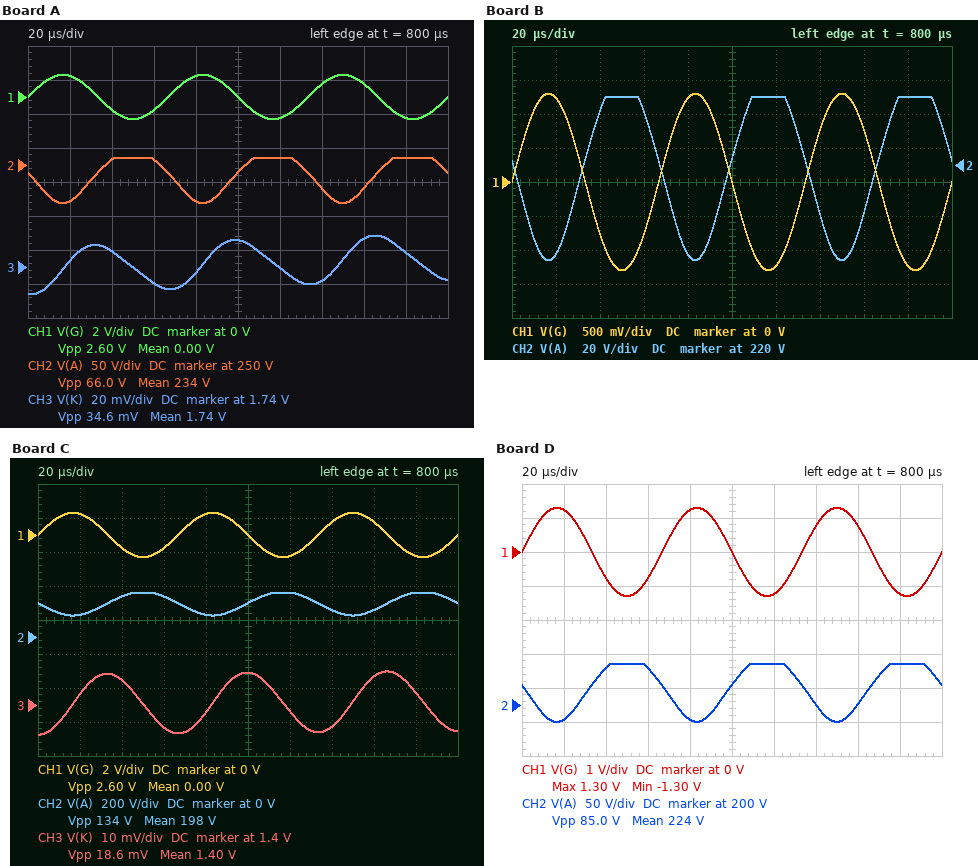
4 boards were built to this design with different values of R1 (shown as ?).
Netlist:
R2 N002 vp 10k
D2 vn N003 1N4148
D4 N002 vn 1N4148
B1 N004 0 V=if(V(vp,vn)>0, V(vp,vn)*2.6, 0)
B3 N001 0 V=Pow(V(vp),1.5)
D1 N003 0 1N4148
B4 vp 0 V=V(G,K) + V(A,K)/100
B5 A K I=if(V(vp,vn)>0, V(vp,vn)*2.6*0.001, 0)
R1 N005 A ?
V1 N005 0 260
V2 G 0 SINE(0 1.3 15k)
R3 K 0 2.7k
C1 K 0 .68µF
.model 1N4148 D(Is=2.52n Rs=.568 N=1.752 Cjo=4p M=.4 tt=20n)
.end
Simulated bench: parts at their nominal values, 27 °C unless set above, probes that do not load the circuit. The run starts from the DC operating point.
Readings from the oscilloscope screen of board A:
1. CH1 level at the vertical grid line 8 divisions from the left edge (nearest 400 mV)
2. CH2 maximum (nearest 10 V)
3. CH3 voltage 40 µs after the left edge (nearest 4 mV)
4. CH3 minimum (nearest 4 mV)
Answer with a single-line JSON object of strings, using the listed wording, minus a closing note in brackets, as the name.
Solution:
{"CH1 level at the vertical grid line 8 divisions from the left edge": "800 mV", "CH2 maximum": "260 V", "CH3 voltage 40 µs after the left edge": "1.748 V", "CH3 minimum": "1.724 V"}
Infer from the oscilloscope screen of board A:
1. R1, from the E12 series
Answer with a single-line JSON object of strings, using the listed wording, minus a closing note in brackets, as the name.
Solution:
{"R1, from the E12 series": "39 kΩ"}
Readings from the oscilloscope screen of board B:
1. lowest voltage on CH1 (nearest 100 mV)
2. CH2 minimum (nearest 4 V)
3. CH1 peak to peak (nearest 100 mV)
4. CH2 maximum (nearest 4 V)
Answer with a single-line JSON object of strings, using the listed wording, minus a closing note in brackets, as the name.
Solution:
{"lowest voltage on CH1": "-1.3 V", "CH2 minimum": "164 V", "CH1 peak to peak": "2.6 V", "CH2 maximum": "260 V"}
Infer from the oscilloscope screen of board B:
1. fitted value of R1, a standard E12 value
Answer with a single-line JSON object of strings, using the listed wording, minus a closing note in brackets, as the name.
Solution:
{"fitted value of R1, a standard E12 value": "68 kΩ"}
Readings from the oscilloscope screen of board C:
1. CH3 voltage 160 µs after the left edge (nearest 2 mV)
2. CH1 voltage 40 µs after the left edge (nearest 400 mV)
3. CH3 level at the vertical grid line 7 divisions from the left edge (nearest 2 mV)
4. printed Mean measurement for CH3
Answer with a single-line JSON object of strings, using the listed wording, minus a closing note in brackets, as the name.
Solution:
{"CH3 voltage 160 µs after the left edge": "1.408 V", "CH1 voltage 40 µs after the left edge": "-800 mV", "CH3 level at the vertical grid line 7 divisions from the left edge": "1.394 V", "printed Mean measurement for CH3": "1.40 V"}
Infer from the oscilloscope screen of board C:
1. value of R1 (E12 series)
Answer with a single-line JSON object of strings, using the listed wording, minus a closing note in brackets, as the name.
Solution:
{"value of R1": "120 kΩ"}
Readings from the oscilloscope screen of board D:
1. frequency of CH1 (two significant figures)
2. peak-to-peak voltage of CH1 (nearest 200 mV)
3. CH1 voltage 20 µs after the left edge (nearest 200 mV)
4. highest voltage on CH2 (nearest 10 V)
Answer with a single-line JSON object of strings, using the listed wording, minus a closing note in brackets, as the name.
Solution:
{"frequency of CH1": "15 kHz", "peak-to-peak voltage of CH1": "2.6 V", "CH1 voltage 20 µs after the left edge": "1.2 V", "highest voltage on CH2": "260 V"}
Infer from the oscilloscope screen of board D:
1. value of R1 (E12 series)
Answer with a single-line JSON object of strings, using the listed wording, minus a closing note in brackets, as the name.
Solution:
{"value of R1": "56 kΩ"}
